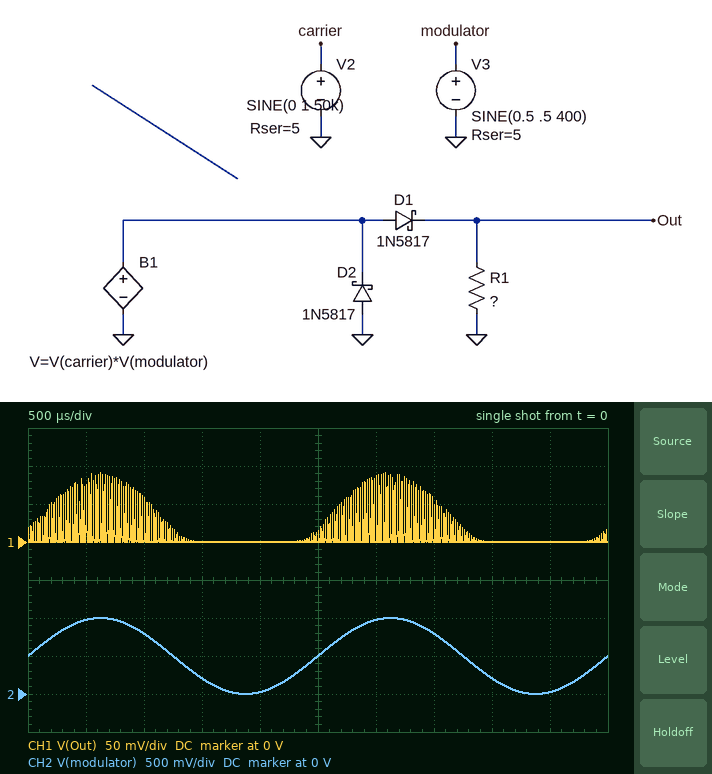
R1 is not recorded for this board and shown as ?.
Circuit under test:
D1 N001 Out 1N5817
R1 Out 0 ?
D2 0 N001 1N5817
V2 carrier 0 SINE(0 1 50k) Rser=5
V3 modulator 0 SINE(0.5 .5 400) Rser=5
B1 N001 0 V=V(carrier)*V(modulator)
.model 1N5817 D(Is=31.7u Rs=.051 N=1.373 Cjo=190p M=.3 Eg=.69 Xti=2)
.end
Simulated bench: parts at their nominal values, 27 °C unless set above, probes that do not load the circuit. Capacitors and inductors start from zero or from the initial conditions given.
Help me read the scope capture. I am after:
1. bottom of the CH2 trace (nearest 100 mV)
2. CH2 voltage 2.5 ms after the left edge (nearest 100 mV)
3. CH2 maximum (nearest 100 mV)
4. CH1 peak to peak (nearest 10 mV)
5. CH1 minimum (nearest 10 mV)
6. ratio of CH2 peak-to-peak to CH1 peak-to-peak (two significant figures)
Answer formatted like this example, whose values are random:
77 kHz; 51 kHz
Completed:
0 V; 500 mV; 1.0 V; 90 mV; 0 V; 11
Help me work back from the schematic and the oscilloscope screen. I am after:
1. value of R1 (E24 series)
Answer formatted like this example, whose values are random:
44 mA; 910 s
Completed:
0.01 Ω
